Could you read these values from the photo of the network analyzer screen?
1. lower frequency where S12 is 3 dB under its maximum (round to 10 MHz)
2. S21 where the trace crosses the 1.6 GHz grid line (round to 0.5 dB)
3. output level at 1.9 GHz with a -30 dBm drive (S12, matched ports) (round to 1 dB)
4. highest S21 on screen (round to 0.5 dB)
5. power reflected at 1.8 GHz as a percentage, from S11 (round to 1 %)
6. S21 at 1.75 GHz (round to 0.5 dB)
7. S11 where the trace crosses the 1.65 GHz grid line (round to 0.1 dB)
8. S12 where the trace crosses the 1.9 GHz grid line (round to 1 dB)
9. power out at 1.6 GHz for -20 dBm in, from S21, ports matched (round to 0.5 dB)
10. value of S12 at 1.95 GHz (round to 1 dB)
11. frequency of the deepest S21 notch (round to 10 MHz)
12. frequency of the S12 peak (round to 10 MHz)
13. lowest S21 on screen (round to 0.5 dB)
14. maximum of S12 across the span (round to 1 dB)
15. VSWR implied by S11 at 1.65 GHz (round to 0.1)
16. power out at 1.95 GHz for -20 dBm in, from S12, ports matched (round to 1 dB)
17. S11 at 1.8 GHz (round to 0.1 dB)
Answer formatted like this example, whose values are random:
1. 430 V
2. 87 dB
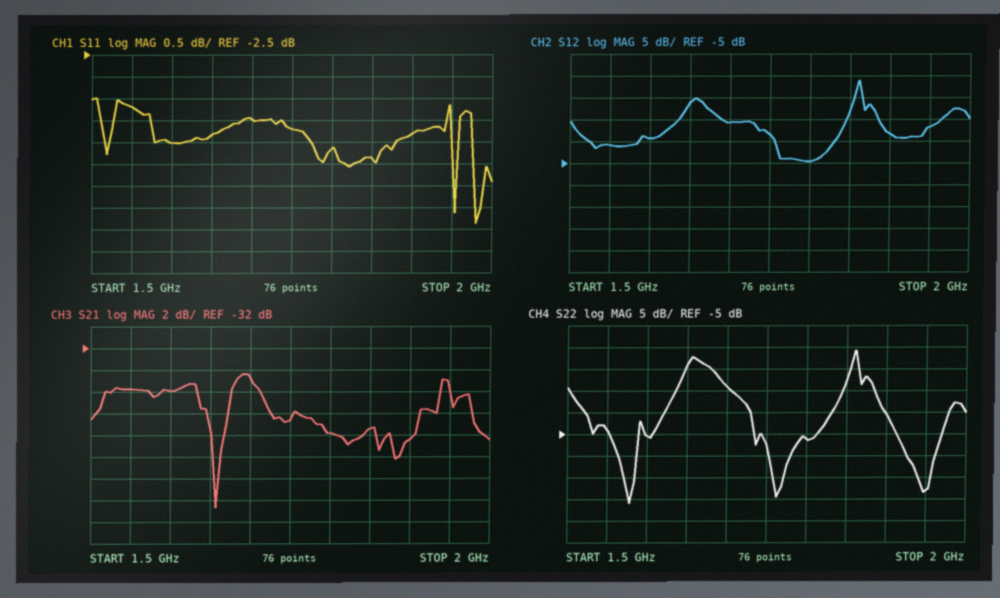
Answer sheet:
1. 1.86 GHz
2. -36.0 dB
3. -28 dBm
4. -34.5 dB
5. 34 %
6. -38.5 dB
7. -4.3 dB
8. 2 dB
9. -56.0 dBm
10. 3 dB
11. 1.66 GHz
12. 1.86 GHz
13. -46.5 dB
14. 14 dB
15. 4.1
16. -17 dBm
17. -4.7 dB
